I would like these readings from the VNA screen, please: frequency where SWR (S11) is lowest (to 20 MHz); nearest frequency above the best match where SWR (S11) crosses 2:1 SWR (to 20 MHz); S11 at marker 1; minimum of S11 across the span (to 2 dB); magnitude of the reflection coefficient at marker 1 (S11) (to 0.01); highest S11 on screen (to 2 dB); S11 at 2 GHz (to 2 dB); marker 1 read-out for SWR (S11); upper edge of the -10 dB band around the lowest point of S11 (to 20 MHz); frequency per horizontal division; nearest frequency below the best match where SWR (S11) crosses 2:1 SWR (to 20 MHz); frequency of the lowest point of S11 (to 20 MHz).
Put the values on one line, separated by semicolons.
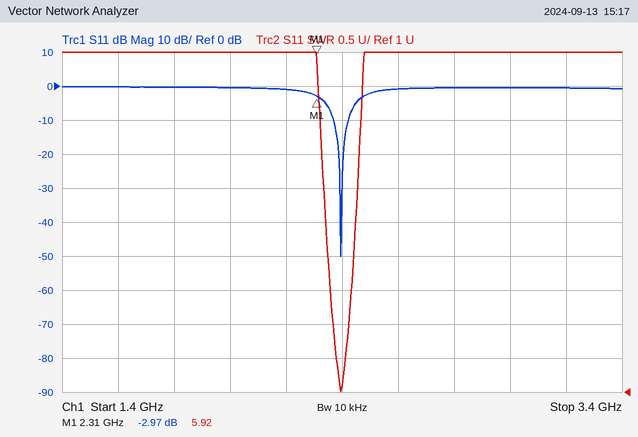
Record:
2.40 GHz; 2.42 GHz; -2.97 dB; -50 dB; 0.71; 0 dB; 0 dB; 5.92; 2.42 GHz; 200 MHz; 2.36 GHz; 2.40 GHz
